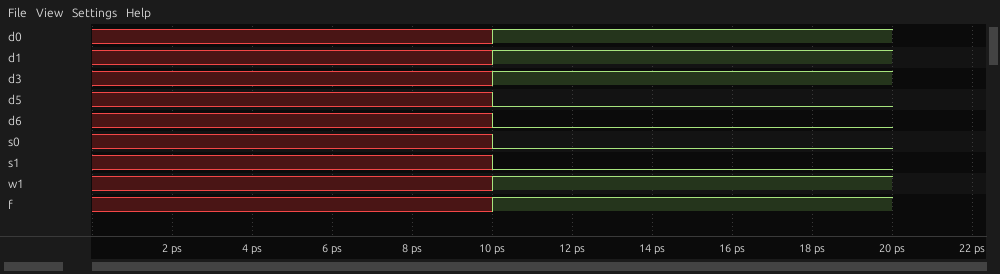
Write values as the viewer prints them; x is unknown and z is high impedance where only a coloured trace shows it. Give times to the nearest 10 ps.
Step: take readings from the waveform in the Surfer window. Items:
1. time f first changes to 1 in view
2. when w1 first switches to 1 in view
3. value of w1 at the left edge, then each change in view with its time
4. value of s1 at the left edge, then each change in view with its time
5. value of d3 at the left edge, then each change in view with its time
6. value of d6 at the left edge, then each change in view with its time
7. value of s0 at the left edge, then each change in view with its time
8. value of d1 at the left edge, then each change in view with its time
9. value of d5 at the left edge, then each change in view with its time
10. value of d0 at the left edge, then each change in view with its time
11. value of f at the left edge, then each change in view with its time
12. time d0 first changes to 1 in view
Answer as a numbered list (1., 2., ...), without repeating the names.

1. 10 ps
2. 10 ps
3. x, 1 at 10 ps
4. x, 0 at 10 ps
5. x, 1 at 10 ps
6. x, 0 at 10 ps
7. x, 0 at 10 ps
8. x, 1 at 10 ps
9. x, 0 at 10 ps
10. x, 1 at 10 ps
11. x, 1 at 10 ps
12. 10 ps
